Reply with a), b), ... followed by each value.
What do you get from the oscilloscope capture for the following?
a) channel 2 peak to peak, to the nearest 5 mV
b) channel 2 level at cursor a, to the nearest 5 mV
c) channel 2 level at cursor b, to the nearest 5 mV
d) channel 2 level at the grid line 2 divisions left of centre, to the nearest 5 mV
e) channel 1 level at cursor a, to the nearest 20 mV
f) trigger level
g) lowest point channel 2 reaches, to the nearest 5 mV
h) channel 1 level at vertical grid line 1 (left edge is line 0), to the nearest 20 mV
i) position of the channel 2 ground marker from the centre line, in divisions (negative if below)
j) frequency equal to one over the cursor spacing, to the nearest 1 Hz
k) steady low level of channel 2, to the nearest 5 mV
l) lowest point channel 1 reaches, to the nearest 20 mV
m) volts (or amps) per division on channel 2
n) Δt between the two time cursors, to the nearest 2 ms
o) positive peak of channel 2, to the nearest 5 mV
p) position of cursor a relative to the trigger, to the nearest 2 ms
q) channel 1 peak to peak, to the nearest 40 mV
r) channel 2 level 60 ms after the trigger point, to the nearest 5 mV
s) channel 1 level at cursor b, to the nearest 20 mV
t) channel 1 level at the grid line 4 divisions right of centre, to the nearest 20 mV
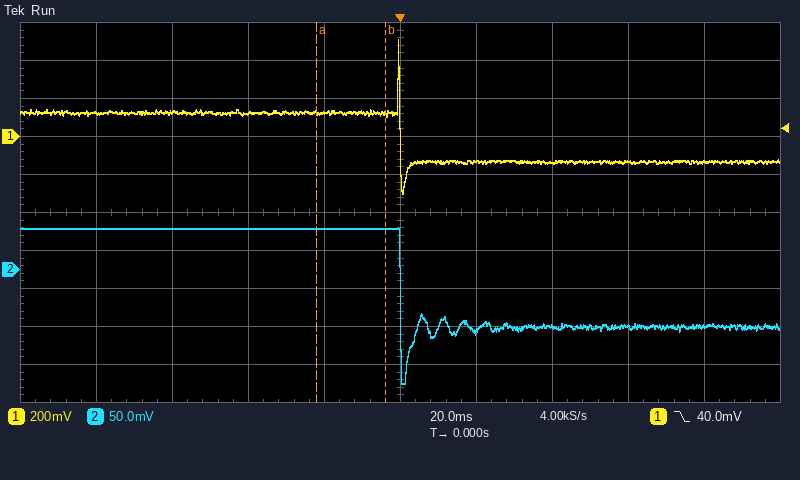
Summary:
a) 205 mV
b) 55 mV
c) 55 mV
d) 55 mV
e) 120 mV
f) 40.0 mV
g) -150 mV
h) 120 mV
i) -1.5 div
j) 56 Hz
k) -75 mV
l) -300 mV
m) 50 mV
n) 18 ms
o) 55 mV
p) -22 ms
q) 800 mV
r) -75 mV
s) 120 mV
t) -140 mV
